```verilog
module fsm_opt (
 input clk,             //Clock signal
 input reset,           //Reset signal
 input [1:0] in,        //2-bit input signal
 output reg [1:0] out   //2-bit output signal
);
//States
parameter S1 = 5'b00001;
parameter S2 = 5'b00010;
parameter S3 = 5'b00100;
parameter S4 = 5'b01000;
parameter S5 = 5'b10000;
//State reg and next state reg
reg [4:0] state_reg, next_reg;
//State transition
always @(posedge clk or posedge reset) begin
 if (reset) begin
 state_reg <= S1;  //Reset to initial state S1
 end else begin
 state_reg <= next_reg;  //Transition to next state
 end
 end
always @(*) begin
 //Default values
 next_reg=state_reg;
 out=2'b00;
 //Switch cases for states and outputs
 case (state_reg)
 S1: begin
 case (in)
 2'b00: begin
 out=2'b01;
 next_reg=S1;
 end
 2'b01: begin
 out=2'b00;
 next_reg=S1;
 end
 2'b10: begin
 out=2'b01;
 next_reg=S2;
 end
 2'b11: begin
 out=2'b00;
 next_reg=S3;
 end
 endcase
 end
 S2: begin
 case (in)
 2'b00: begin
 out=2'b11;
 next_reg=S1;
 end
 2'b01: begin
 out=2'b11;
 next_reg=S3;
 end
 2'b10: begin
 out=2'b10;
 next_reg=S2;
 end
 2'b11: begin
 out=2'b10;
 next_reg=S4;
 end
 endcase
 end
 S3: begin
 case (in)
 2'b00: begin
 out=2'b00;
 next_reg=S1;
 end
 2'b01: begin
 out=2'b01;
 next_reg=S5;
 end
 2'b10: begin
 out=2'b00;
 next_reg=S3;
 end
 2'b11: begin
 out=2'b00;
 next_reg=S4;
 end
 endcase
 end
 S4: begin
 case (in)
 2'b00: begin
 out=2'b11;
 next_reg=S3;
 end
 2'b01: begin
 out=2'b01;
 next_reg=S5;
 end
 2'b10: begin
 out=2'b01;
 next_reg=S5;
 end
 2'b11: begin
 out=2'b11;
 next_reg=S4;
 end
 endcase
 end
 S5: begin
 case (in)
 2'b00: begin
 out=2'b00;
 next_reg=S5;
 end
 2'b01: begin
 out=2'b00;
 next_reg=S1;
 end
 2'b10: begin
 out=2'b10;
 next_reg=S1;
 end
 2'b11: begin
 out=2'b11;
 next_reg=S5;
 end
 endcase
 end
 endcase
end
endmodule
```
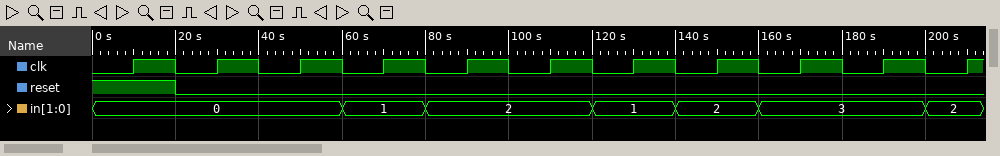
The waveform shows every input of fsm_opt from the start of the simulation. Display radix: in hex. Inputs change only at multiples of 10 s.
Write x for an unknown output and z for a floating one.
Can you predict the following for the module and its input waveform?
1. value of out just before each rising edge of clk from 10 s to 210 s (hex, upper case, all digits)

1, 1, 1, 0, 1, 2, 3, 0, 0, 3, 1
